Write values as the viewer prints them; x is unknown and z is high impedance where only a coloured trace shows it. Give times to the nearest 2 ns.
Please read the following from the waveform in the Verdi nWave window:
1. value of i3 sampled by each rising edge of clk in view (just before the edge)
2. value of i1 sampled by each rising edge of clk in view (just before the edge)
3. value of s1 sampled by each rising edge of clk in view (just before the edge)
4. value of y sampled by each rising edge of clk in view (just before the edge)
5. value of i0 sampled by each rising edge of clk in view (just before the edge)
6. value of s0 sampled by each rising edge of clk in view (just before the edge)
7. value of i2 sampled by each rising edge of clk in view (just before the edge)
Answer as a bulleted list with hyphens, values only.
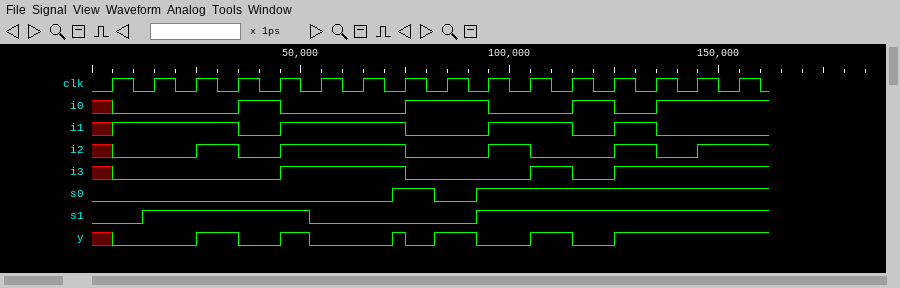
- x 0 0 0 0 1 1 1 0 0 0 1 0 1 1 1
- x 1 1 1 0 1 1 1 0 0 1 1 0 1 0 0
- 0 1 1 1 1 0 0 0 0 1 1 1 1 1 1 1
- x 0 0 1 0 0 0 1 1 0 0 1 0 1 1 1
- x 0 0 0 1 0 0 0 1 1 0 0 1 0 1 1
- 0 0 0 0 0 0 0 1 0 1 1 1 1 1 1 1
- x 0 0 1 0 1 1 1 0 0 1 0 0 1 0 1
